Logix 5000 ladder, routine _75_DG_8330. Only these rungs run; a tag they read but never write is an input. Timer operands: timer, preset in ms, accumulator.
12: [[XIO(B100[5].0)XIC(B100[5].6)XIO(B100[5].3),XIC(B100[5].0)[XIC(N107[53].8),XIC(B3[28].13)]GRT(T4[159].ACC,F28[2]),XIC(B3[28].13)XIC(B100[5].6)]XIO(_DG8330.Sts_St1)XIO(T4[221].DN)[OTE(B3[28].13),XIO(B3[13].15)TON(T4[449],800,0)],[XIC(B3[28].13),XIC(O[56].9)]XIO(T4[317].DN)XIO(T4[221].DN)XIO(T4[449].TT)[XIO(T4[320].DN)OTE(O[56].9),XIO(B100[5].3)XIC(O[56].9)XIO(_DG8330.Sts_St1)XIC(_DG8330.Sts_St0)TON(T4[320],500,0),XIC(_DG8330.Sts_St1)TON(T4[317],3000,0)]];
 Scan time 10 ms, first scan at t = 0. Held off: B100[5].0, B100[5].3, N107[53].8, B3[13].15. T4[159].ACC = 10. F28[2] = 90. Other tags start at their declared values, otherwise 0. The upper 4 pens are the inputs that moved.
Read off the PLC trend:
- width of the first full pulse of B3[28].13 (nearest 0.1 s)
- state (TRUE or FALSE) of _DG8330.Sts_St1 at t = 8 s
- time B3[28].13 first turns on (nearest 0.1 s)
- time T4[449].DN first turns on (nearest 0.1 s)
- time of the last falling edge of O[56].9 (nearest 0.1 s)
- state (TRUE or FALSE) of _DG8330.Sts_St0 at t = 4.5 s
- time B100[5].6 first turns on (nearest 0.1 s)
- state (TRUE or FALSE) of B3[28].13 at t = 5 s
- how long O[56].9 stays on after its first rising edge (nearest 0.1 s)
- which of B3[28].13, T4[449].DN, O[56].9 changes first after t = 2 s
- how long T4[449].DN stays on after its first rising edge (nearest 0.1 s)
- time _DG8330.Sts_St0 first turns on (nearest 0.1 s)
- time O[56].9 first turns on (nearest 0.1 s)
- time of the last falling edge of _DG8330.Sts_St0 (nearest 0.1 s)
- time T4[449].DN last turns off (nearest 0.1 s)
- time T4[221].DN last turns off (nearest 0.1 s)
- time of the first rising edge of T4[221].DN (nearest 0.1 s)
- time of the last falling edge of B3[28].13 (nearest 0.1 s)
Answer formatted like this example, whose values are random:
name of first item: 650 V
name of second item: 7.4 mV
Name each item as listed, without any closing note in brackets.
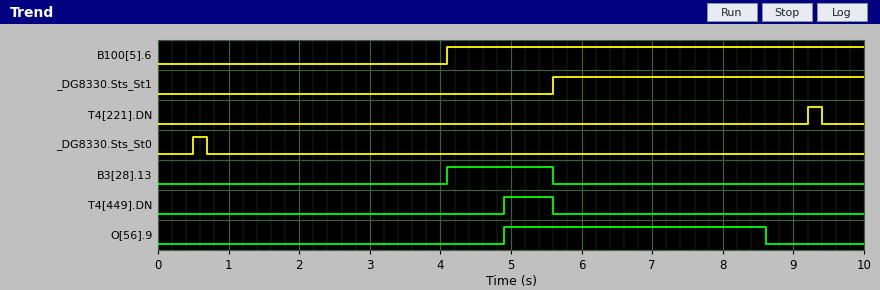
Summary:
width of the first full pulse of B3[28].13: 1.5 s
state (TRUE or FALSE) of _DG8330.Sts_St1 at t = 8 s: TRUE
time B3[28].13 first turns on: 4.1 s
time T4[449].DN first turns on: 4.9 s
time of the last falling edge of O[56].9: 8.6 s
state (TRUE or FALSE) of _DG8330.Sts_St0 at t = 4.5 s: FALSE
time B100[5].6 first turns on: 4.1 s
state (TRUE or FALSE) of B3[28].13 at t = 5 s: TRUE
how long O[56].9 stays on after its first rising edge: 3.7 s
which of B3[28].13, T4[449].DN, O[56].9 changes first after t = 2 s: B3[28].13
how long T4[449].DN stays on after its first rising edge: 0.7 s
time _DG8330.Sts_St0 first turns on: 0.5 s
time O[56].9 first turns on: 4.9 s
time of the last falling edge of _DG8330.Sts_St0: 0.7 s
time T4[449].DN last turns off: 5.6 s
time T4[221].DN last turns off: 9.4 s
time of the first rising edge of T4[221].DN: 9.2 s
time of the last falling edge of B3[28].13: 5.6 s
